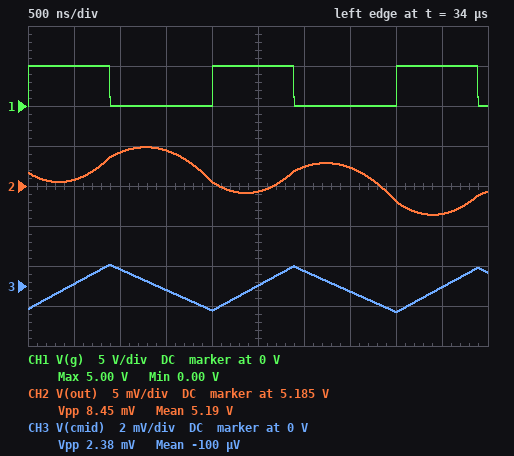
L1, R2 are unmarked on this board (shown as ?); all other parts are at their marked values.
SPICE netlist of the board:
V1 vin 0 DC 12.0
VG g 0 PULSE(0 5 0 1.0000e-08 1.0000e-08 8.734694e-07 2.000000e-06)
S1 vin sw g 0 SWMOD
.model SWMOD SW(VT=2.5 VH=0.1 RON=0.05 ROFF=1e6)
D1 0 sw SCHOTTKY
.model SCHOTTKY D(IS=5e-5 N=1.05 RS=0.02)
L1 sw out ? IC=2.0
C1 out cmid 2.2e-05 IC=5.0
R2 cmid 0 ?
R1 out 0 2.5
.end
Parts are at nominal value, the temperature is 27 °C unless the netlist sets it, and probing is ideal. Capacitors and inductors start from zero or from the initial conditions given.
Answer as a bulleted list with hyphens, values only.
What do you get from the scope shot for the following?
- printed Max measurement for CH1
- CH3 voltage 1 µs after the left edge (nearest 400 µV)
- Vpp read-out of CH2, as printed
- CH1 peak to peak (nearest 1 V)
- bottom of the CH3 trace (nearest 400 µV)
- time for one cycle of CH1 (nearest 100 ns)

- 5.00 V
- 800 µV
- 8.45 mV
- 5 V
- -1.2 mV
- 2.0 µs
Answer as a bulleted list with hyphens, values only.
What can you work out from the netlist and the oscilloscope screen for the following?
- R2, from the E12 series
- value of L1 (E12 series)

- 5.6 mΩ
- 15 µH
